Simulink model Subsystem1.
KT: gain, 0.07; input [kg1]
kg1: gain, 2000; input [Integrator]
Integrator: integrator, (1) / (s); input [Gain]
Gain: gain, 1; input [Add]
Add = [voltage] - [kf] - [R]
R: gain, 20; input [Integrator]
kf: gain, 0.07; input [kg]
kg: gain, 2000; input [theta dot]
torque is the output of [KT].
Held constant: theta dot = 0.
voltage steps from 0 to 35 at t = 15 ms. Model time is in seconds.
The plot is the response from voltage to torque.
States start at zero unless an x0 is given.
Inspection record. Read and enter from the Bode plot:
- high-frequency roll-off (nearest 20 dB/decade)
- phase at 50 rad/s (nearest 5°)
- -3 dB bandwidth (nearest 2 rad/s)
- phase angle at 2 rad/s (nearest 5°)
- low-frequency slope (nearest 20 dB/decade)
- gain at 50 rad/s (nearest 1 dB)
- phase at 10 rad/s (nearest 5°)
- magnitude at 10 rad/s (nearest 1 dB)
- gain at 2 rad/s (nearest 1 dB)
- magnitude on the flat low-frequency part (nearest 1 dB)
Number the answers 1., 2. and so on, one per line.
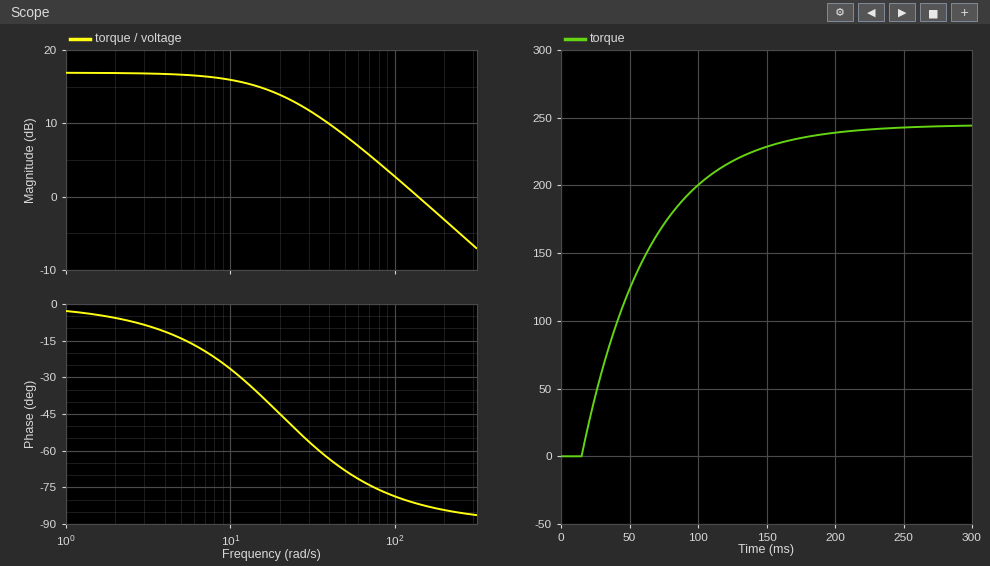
1. -20 dB/decade
2. -70°
3. 20 rad/s
4. -5°
5. 0 dB/decade
6. 8 dB
7. -25°
8. 16 dB
9. 17 dB
10. 17 dB
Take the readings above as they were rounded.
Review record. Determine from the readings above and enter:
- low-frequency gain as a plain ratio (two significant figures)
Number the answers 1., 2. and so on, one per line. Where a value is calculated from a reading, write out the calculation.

1. 10^(17 / 20) = 7.1
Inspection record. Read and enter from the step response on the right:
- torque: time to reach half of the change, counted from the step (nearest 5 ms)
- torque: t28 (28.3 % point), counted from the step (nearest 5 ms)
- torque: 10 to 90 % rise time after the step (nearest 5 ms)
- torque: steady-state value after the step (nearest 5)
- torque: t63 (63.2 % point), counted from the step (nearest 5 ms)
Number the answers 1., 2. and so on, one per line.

1. 35 ms
2. 15 ms
3. 110 ms
4. 245
5. 50 ms
